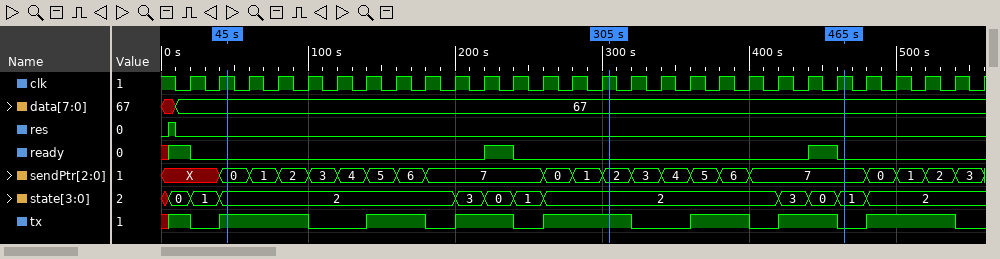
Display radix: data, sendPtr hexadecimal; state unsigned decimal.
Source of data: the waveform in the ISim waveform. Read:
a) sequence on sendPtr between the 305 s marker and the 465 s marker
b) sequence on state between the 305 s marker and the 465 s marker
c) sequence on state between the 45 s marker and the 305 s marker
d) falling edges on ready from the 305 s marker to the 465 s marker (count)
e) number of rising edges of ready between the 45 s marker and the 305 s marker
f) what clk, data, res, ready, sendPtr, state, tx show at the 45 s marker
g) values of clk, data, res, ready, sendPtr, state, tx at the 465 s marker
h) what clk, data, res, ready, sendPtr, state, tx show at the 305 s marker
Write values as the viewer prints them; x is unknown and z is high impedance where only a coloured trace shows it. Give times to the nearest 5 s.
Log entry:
2, 3, 4, 5, 6, 7
2, 3, 0, 1
2, 3, 0, 1, 2
1
1
clk=1, data=67, res=0, ready=0, sendPtr=0, state=2, tx=1
clk=1, data=67, res=0, ready=0, sendPtr=7, state=1, tx=0
clk=1, data=67, res=0, ready=0, sendPtr=2, state=2, tx=1
